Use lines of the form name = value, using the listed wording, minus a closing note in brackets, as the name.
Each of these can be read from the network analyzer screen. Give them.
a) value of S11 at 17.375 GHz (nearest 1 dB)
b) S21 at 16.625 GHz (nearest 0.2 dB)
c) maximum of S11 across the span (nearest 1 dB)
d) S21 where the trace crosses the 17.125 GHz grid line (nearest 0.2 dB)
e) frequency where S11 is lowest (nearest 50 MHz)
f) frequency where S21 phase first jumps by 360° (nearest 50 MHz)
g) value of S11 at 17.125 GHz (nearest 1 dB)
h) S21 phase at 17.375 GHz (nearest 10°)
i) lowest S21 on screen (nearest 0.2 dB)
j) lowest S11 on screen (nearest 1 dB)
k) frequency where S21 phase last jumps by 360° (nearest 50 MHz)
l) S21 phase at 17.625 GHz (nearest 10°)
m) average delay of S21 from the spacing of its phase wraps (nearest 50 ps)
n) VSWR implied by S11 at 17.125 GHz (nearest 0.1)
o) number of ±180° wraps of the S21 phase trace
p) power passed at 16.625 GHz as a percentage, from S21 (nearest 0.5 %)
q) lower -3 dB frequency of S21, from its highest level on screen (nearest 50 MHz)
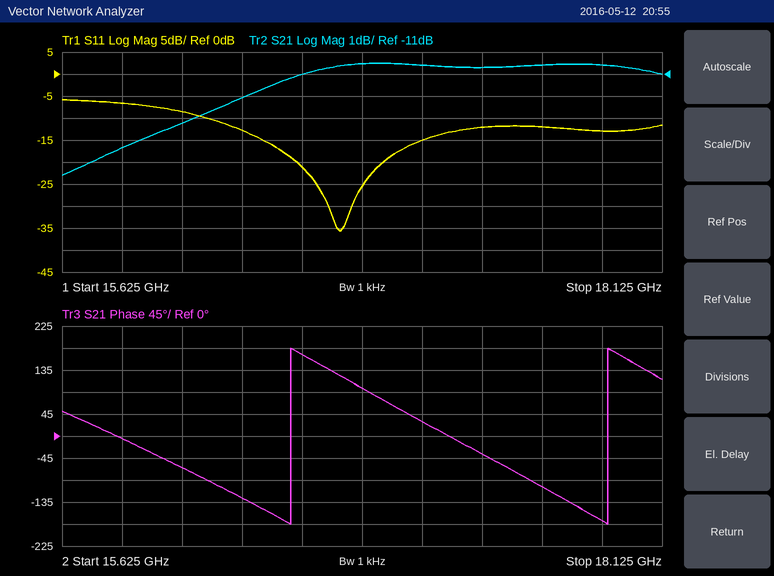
value of S11 at 17.375 GHz = -12 dB
S21 at 16.625 GHz = -11.0 dB
maximum of S11 across the span = -6 dB
S21 where the trace crosses the 17.125 GHz grid line = -10.6 dB
frequency where S11 is lowest = 16.80 GHz
frequency where S21 phase first jumps by 360° = 16.60 GHz
value of S11 at 17.125 GHz = -15 dB
S21 phase at 17.375 GHz = -40°
lowest S21 on screen = -15.6 dB
lowest S11 on screen = -36 dB
frequency where S21 phase last jumps by 360° = 17.90 GHz
S21 phase at 17.625 GHz = -100°
average delay of S21 from the spacing of its phase wraps = 750 ps
VSWR implied by S11 at 17.125 GHz = 1.4
number of ±180° wraps of the S21 phase trace = 2
power passed at 16.625 GHz as a percentage, from S21 = 8.0 %
lower -3 dB frequency of S21, from its highest level on screen = 16.05 GHz
